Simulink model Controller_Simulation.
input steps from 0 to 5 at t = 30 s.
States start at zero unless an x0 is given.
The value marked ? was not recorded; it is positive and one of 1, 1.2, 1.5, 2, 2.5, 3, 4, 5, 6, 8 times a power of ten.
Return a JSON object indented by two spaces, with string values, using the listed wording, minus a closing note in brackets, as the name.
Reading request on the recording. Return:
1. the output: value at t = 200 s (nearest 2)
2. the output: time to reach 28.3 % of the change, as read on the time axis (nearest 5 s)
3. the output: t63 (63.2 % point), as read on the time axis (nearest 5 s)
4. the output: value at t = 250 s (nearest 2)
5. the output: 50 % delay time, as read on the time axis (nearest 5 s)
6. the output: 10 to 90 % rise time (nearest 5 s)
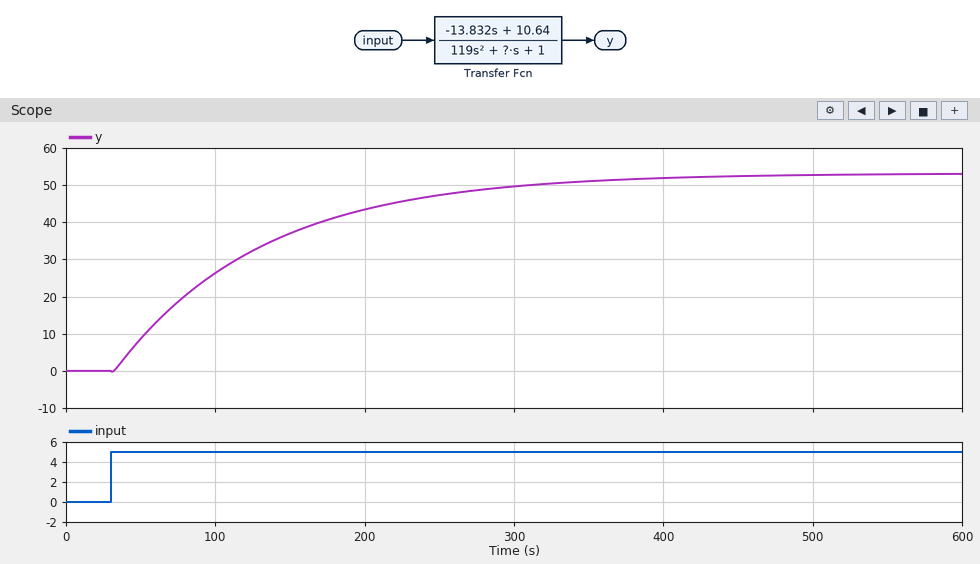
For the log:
{
  "the output: value at t = 200 s": "44",
  "the output: time to reach 28.3 % of the change, as read on the time axis": "65 s",
  "the output: t63 (63.2 % point), as read on the time axis": "130 s",
  "the output: value at t = 250 s": "48",
  "the output: 50 % delay time, as read on the time axis": "100 s",
  "the output: 10 to 90 % rise time": "215 s"
}
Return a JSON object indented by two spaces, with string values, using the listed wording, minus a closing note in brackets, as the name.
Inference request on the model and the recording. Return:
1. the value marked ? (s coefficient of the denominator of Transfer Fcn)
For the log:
{
  "the value marked ?": "100"
}
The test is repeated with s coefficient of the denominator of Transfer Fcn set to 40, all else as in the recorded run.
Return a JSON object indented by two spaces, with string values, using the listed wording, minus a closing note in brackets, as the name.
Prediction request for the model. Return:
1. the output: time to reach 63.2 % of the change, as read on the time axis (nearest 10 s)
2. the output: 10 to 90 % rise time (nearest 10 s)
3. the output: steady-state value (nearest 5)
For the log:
{
  "the output: time to reach 63.2 % of the change, as read on the time axis": "70 s",
  "the output: 10 to 90 % rise time": "80 s",
  "the output: steady-state value": "55"
}
